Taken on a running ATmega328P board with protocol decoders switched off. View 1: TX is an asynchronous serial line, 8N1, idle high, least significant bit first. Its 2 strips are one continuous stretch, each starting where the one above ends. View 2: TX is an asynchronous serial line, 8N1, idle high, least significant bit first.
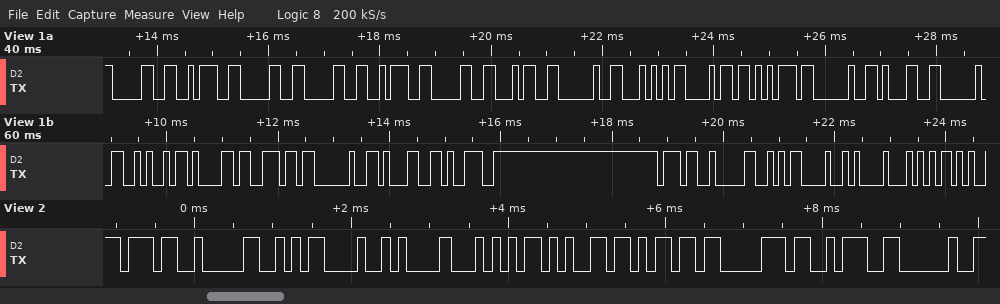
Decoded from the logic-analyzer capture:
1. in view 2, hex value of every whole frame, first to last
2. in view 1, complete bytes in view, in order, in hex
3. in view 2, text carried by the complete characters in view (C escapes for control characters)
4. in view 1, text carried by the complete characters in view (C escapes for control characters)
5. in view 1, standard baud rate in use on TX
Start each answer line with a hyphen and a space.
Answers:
- 37 30 0D 0A 54 65 6D 70 3A 20
- 30 3A 30 30 3A 30 34 20 54 68 75 20 31 20 4A 61 6E 20 31 39 37 30 0D 0A 54
- "70\r\nTemp: "
- "0:00:04 Thu 1 Jan 1970\r\nT"
- 9600 baud
